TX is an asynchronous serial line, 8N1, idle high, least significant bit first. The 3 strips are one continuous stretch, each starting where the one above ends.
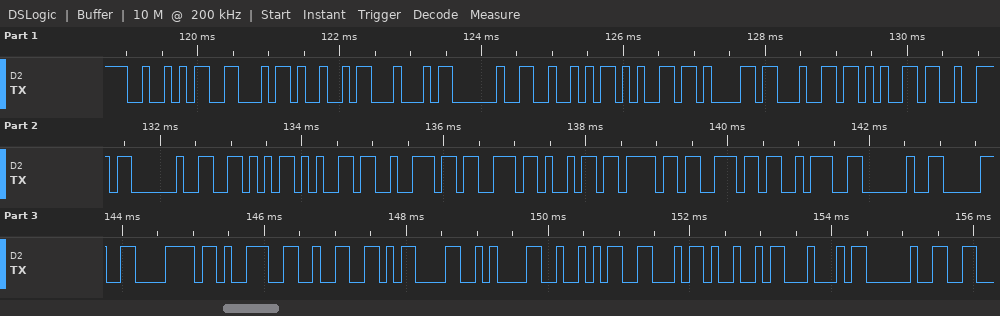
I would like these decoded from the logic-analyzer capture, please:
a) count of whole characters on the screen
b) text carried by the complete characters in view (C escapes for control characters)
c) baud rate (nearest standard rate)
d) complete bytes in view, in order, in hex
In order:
32
"RFID Reader Version: 0x92\r\nRFID "
9600 baud
52 46 49 44 20 52 65 61 64 65 72 20 56 65 72 73 69 6F 6E 3A 20 30 78 39 32 0D 0A 52 46 49 44 20
